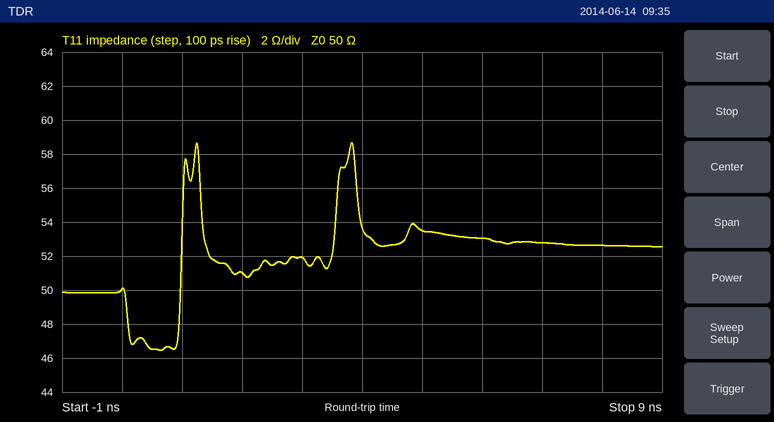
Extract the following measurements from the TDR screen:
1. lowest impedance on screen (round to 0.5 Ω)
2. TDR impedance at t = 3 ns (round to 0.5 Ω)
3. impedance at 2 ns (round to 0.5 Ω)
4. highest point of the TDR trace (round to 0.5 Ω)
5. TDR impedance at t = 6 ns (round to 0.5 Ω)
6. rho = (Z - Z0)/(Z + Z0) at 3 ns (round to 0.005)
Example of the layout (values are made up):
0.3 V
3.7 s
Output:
46.5 Ω
52.0 Ω
51.0 Ω
58.5 Ω
53.0 Ω
+0.020
